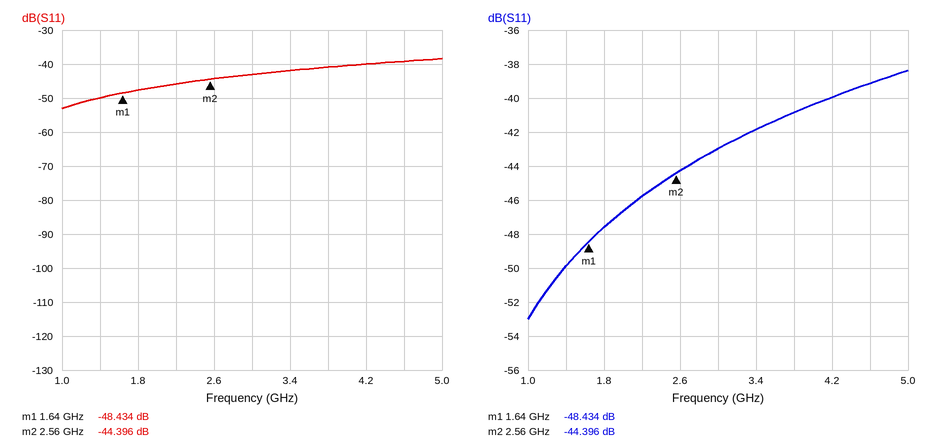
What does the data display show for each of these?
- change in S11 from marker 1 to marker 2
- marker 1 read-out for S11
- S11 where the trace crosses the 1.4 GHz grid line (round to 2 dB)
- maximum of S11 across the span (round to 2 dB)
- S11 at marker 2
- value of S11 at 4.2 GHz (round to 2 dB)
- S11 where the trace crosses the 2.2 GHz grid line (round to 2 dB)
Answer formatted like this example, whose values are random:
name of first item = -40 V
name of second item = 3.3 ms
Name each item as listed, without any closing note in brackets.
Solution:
change in S11 from marker 1 to marker 2 = 4.038 dB
marker 1 read-out for S11 = -48.434 dB
S11 where the trace crosses the 1.4 GHz grid line = -50 dB
maximum of S11 across the span = -38 dB
S11 at marker 2 = -44.396 dB
value of S11 at 4.2 GHz = -40 dB
S11 where the trace crosses the 2.2 GHz grid line = -46 dB
